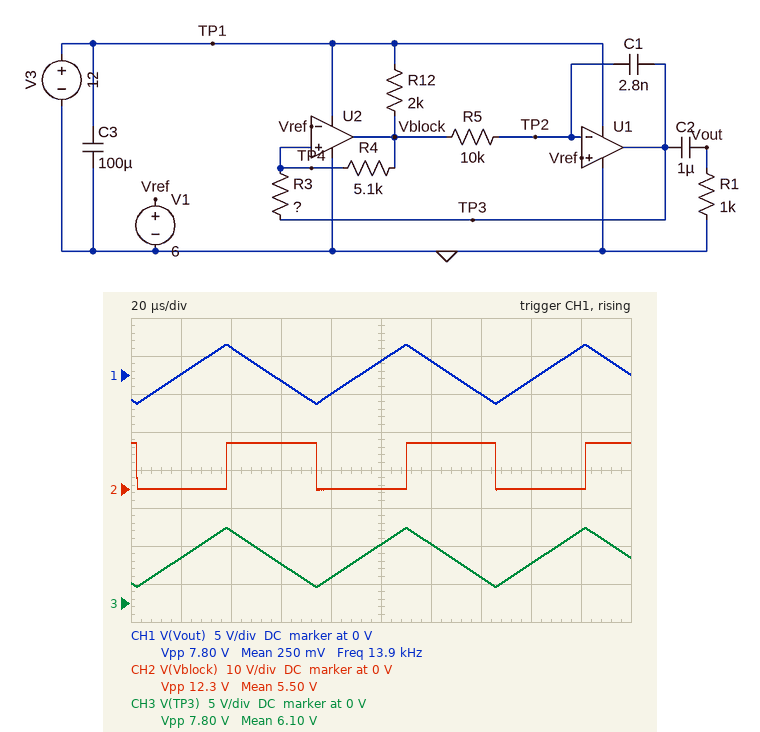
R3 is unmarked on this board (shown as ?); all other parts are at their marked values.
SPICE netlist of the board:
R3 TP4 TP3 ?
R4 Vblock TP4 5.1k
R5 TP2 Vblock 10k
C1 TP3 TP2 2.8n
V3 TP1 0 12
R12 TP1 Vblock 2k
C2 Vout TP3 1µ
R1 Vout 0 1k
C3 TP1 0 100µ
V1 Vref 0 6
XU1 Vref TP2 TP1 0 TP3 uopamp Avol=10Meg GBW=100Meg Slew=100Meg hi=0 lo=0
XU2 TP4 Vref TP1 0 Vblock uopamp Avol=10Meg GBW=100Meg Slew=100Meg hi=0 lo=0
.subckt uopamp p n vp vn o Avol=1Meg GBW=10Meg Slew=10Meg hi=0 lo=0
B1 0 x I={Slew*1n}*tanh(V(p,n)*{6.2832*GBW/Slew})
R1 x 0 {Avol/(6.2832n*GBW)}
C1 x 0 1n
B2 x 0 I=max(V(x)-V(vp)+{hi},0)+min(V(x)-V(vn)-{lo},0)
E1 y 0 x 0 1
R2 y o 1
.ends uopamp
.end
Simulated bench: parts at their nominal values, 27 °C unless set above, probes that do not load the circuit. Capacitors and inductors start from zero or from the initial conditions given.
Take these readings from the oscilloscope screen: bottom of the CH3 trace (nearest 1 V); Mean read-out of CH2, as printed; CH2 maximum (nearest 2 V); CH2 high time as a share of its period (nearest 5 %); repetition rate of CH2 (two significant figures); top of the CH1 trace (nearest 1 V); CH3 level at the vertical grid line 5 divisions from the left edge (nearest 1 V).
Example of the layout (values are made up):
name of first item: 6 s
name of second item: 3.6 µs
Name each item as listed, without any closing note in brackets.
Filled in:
bottom of the CH3 trace: 2 V
Mean read-out of CH2, as printed: 5.50 V
CH2 maximum: 12 V
CH2 high time as a share of its period: 50 %
repetition rate of CH2: 14 kHz
top of the CH1 trace: 4 V
CH3 level at the vertical grid line 5 divisions from the left edge: 8 V
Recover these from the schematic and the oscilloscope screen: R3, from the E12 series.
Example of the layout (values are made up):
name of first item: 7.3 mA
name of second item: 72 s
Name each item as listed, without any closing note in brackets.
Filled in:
R3, from the E12 series: 3.3 kΩ
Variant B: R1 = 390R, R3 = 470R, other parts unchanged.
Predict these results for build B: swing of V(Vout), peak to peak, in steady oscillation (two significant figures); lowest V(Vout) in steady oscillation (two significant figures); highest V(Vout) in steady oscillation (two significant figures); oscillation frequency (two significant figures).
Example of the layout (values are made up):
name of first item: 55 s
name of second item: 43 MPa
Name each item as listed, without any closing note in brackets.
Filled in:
swing of V(Vout), peak to peak, in steady oscillation: 1.1 V
lowest V(Vout) in steady oscillation: -570 mV
highest V(Vout) in steady oscillation: 570 mV
oscillation frequency: 94 kHz
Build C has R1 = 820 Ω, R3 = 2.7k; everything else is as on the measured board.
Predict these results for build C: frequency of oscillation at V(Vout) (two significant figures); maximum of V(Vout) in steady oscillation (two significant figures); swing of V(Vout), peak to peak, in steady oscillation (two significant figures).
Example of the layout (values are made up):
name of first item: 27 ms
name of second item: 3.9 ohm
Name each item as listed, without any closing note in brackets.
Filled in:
frequency of oscillation at V(Vout): 17 kHz
maximum of V(Vout) in steady oscillation: 3.2 V
swing of V(Vout), peak to peak, in steady oscillation: 6.4 V
